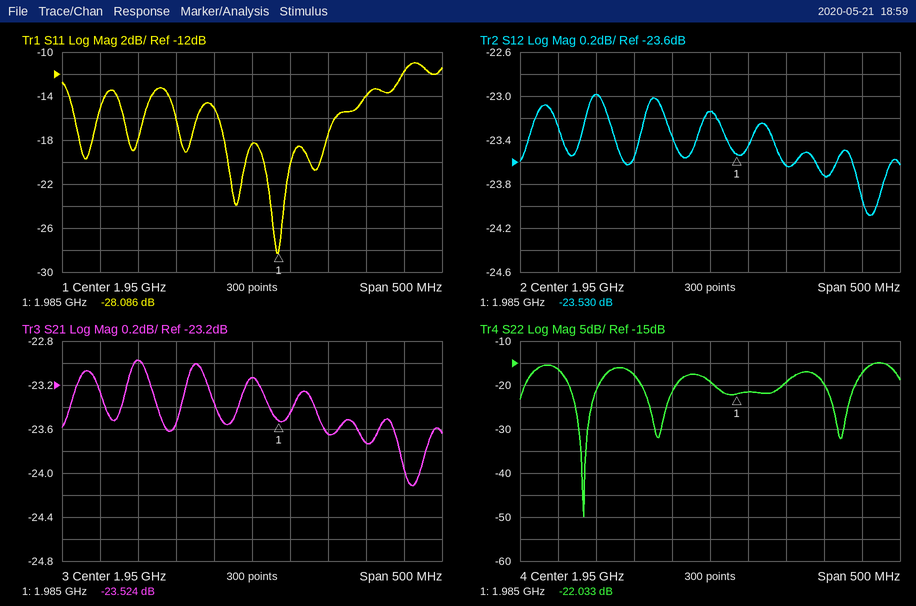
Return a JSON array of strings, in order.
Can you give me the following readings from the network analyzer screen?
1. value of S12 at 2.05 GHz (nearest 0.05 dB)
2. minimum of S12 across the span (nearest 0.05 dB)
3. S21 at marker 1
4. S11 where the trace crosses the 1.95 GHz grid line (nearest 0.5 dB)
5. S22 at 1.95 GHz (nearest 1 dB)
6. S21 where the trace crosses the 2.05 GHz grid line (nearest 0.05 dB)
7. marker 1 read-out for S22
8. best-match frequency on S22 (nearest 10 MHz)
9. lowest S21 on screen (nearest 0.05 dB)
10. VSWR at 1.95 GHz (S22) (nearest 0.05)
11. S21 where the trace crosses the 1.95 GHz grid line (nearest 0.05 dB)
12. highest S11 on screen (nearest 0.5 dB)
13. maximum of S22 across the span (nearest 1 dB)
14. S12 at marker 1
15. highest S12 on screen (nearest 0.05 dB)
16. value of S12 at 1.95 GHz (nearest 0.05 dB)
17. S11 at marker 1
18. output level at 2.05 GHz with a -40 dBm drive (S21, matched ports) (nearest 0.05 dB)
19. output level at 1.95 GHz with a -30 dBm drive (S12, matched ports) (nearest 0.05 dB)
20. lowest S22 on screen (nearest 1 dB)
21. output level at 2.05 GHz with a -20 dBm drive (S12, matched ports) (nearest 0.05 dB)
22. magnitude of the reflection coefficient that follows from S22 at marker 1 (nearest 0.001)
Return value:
["-23.65 dB", "-24.10 dB", "-23.524 dB", "-18.5 dB", "-19 dB", "-23.65 dB", "-22.033 dB", "1.78 GHz", "-24.10 dB", "1.25", "-23.15 dB", "-11.0 dB", "-15 dB", "-23.530 dB", "-23.00 dB", "-23.15 dB", "-28.086 dB", "-63.65 dBm", "-53.15 dBm", "-50 dB", "-43.65 dBm", "0.079"]
